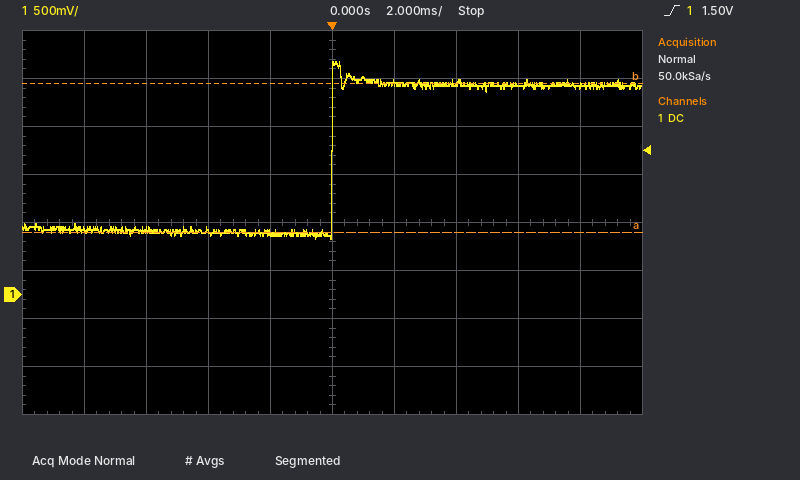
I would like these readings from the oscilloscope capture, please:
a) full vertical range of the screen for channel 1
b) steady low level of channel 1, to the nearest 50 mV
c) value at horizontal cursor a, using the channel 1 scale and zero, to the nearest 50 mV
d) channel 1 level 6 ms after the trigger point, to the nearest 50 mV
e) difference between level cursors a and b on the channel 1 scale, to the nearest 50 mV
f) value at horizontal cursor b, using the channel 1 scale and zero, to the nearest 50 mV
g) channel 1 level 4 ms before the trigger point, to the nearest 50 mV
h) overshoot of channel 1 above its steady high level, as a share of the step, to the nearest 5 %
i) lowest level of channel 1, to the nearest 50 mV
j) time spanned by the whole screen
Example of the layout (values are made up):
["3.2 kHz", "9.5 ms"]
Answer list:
["4 V", "650 mV", "650 mV", "2.20 V", "1.55 V", "2.20 V", "650 mV", "15 %", "600 mV", "20 ms"]
